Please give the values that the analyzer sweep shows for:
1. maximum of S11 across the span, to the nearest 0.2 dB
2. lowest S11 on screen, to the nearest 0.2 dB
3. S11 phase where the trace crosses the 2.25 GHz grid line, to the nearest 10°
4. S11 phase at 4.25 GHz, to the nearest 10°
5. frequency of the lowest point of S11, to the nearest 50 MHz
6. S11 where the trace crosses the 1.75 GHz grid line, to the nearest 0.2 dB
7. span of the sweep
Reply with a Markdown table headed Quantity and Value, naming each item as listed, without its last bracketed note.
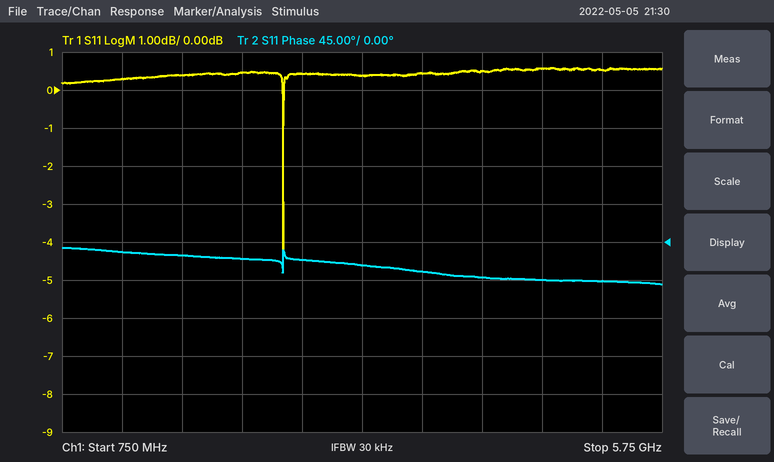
| Quantity | Value |
|---|---|
| maximum of S11 across the span, to the nearest 0.2 dB | 0.6 dB |
| lowest S11 on screen, to the nearest 0.2 dB | -4.2 dB |
| S11 phase where the trace crosses the 2.25 GHz grid line, to the nearest 10° | -20° |
| S11 phase at 4.25 GHz, to the nearest 10° | -40° |
| frequency of the lowest point of S11, to the nearest 50 MHz | 2.60 GHz |
| S11 where the trace crosses the 1.75 GHz grid line, to the nearest 0.2 dB | 0.4 dB |
| span of the sweep | 5 GHz |
